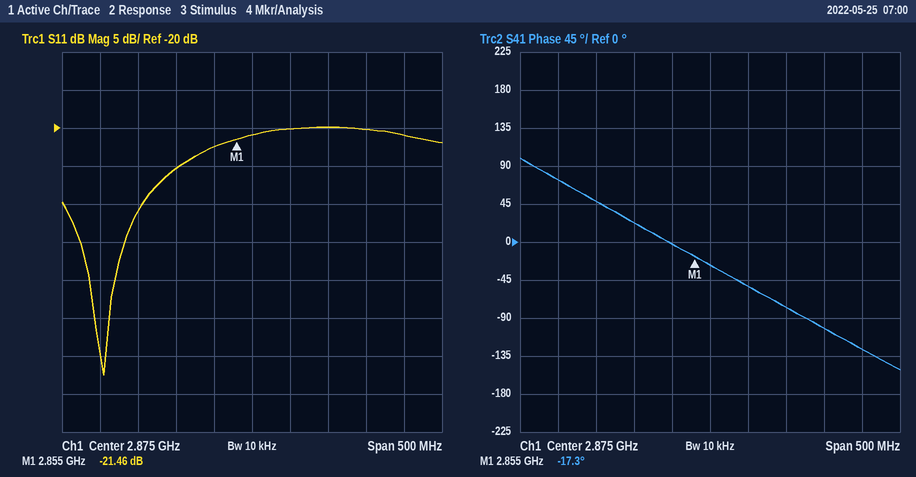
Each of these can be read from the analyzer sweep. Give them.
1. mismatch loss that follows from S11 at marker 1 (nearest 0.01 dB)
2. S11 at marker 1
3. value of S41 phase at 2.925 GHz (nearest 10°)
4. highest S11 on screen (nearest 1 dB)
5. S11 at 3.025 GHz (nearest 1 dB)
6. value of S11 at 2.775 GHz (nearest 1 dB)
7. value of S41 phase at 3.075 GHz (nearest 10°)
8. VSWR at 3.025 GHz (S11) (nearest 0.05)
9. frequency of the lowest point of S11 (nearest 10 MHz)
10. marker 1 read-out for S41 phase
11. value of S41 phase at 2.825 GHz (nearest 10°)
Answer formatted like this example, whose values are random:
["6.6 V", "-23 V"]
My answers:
["0.03 dB", "-21.46 dB", "-50°", "-20 dB", "-20 dB", "-25 dB", "-130°", "1.20", "2.68 GHz", "-17.3°", "0°"]
